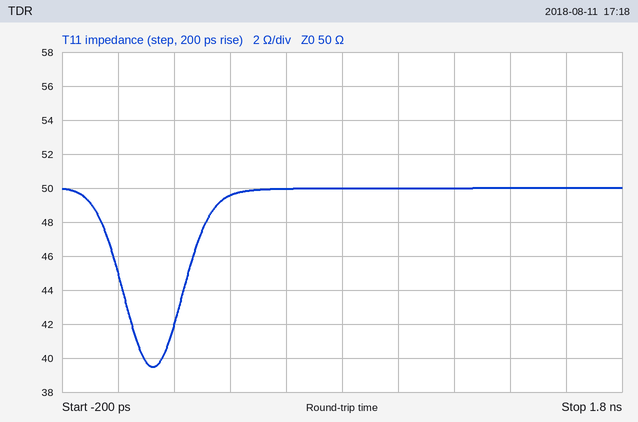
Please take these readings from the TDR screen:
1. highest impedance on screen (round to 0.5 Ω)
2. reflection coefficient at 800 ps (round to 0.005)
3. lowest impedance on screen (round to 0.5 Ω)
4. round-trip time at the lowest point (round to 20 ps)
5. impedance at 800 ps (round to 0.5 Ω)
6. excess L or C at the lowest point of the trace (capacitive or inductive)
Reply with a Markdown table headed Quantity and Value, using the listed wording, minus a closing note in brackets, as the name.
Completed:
| Quantity | Value |
|---|---|
| highest impedance on screen | 50.0 Ω |
| reflection coefficient at 800 ps | 0.000 |
| lowest impedance on screen | 39.5 Ω |
| round-trip time at the lowest point | 120 ps |
| impedance at 800 ps | 50.0 Ω |
| excess L or C at the lowest point of the trace | capacitive |
